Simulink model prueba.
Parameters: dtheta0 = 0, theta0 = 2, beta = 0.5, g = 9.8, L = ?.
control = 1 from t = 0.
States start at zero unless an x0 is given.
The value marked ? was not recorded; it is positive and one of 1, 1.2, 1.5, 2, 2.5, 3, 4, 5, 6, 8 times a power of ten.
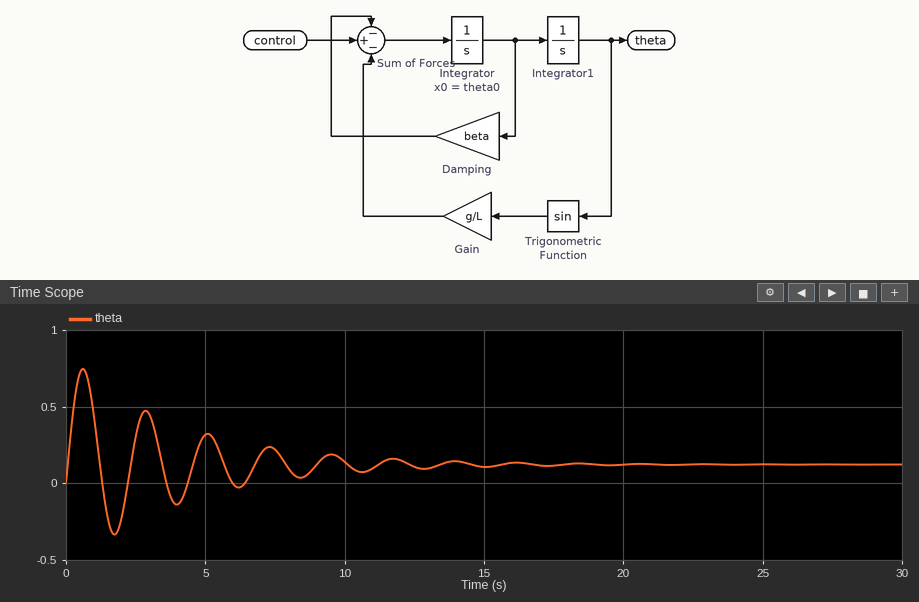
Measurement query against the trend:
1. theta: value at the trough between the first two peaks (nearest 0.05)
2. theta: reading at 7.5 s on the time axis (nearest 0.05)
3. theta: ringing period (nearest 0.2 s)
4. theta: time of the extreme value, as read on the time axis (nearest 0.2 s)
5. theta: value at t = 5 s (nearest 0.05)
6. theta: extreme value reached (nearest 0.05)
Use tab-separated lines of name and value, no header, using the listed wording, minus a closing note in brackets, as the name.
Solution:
theta: value at the trough between the first two peaks	-0.35
theta: reading at 7.5 s on the time axis	0.20
theta: ringing period	2.2 s
theta: time of the extreme value, as read on the time axis	0.6 s
theta: value at t = 5 s	0.30
theta: extreme value reached	0.75
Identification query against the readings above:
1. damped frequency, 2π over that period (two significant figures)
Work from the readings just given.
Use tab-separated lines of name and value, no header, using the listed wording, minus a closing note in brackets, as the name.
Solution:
damped frequency, 2π over that period	2.9 rad/s
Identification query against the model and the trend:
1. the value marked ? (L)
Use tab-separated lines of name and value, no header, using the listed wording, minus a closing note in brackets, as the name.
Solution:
the value marked ?	1.2
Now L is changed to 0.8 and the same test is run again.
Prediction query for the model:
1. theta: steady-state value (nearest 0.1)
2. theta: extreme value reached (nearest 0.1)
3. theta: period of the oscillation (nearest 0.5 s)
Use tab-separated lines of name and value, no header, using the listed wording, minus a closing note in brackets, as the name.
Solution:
theta: steady-state value	0.1
theta: extreme value reached	0.6
theta: period of the oscillation	2.0 s
